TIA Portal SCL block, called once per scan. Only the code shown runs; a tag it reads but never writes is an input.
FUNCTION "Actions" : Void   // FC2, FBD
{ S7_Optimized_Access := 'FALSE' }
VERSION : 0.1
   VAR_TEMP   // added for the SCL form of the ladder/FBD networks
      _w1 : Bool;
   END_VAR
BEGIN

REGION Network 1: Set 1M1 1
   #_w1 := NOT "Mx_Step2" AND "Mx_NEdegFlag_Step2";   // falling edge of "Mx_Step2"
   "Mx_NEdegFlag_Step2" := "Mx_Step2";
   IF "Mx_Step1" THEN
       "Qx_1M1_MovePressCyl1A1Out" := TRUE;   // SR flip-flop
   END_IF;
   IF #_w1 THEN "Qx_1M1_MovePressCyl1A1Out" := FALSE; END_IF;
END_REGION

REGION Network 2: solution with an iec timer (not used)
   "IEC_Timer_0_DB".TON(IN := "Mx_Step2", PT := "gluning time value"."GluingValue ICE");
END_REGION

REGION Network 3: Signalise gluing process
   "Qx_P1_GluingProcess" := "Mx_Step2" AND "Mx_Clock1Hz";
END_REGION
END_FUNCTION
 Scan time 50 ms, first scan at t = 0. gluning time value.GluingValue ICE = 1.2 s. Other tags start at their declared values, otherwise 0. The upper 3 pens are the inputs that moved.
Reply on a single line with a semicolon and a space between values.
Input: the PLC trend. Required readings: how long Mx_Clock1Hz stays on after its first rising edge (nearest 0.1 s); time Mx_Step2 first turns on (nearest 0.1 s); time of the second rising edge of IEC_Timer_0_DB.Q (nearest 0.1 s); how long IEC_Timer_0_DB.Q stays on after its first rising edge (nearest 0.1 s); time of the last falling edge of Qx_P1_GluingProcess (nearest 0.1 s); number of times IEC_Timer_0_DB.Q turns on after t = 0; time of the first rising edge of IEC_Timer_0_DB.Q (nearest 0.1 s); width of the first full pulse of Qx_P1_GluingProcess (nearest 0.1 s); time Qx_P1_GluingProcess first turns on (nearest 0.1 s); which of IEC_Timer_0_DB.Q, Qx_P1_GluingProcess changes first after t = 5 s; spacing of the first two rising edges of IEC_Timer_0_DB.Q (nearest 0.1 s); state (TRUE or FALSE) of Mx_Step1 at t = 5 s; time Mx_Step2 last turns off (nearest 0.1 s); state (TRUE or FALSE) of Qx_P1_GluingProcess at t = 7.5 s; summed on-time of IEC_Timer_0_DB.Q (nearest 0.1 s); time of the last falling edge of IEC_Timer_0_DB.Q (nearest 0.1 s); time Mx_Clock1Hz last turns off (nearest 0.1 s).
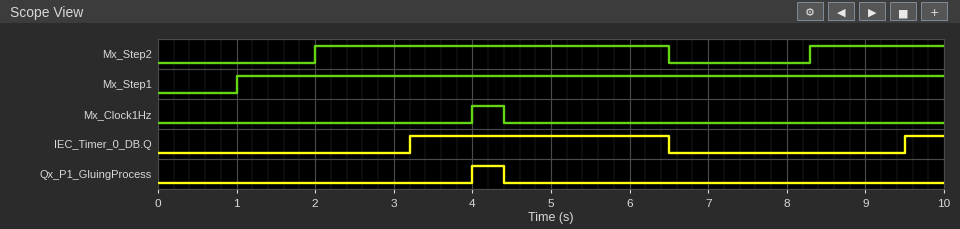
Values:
0.4 s; 2.0 s; 9.5 s; 3.3 s; 4.4 s; 2; 3.2 s; 0.4 s; 4.0 s; IEC_Timer_0_DB.Q; 6.3 s; TRUE; 6.5 s; FALSE; 3.8 s; 6.5 s; 4.4 s
